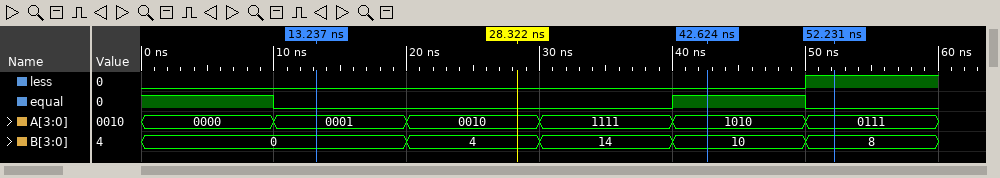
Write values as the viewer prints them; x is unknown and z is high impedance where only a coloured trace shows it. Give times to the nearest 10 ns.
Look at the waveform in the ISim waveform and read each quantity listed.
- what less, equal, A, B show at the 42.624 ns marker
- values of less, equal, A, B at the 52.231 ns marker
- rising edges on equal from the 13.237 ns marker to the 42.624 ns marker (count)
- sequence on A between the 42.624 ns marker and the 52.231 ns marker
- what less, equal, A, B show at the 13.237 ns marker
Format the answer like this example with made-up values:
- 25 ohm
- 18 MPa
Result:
- less=0, equal=1, A=1010, B=10
- less=1, equal=0, A=0111, B=8
- 1
- 1010, 0111
- less=0, equal=0, A=0001, B=0
